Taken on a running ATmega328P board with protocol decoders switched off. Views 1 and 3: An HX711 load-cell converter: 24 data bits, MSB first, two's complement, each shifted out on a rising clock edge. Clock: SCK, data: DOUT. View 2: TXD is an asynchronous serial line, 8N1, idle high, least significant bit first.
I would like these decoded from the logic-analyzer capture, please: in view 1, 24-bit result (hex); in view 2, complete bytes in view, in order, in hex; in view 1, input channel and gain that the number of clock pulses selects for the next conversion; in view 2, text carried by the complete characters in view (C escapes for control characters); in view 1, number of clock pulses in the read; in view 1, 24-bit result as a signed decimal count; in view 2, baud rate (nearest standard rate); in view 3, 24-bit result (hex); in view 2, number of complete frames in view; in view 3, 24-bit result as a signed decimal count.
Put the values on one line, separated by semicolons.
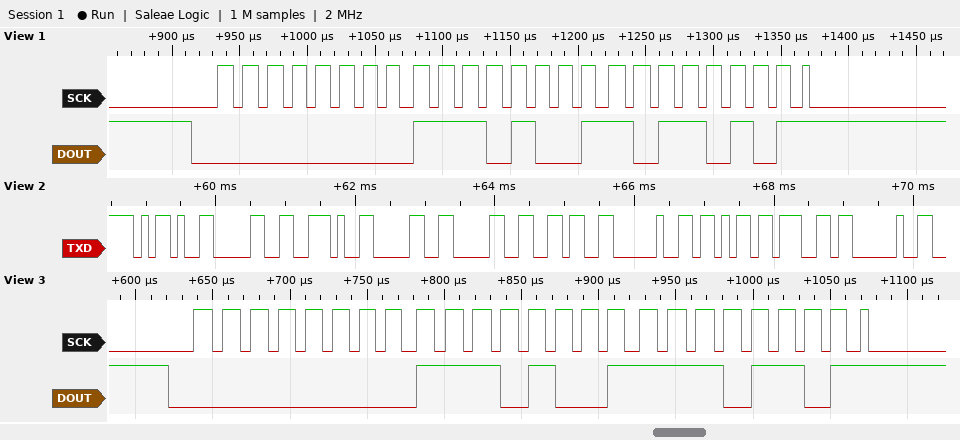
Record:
0x00E9B5; 2D 30 2E 30 30 36 20 6B 67 20; channel A, gain 128; "-0.006 kg "; 25; 59829; 9600 baud; 0x00E9ED; 10; 59885
